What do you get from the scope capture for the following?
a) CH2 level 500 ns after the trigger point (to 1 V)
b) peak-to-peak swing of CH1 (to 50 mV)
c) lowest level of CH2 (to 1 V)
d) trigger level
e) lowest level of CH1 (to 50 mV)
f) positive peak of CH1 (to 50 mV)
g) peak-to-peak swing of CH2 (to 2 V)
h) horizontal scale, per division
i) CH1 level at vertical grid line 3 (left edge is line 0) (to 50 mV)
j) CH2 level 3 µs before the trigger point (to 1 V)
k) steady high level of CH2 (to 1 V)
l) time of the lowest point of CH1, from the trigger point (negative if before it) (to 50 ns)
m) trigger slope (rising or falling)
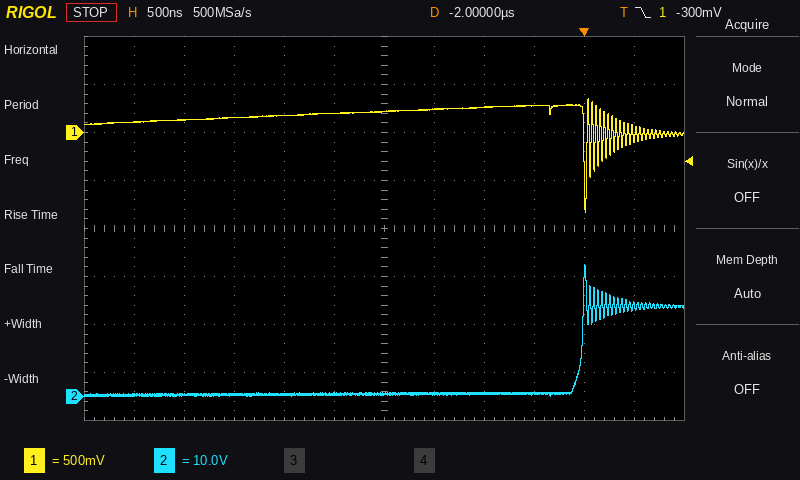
19 V
1.20 V
0 V
-300 mV
-850 mV
350 mV
28 V
500 ns
150 mV
0 V
19 V
0 ns
falling
